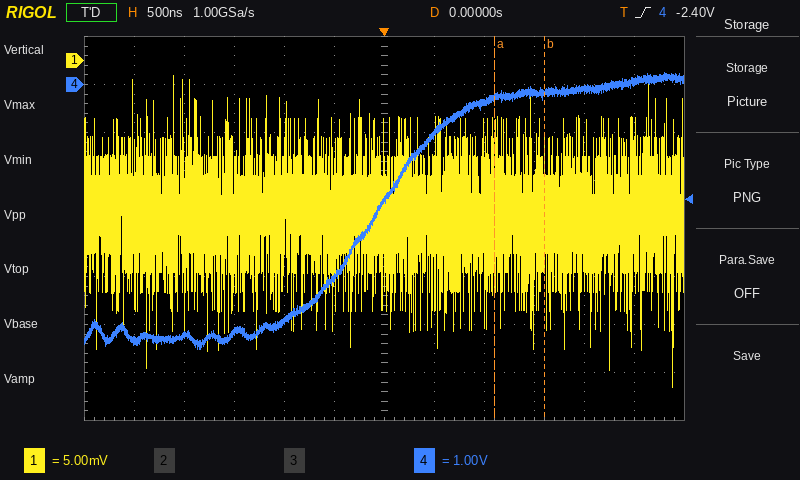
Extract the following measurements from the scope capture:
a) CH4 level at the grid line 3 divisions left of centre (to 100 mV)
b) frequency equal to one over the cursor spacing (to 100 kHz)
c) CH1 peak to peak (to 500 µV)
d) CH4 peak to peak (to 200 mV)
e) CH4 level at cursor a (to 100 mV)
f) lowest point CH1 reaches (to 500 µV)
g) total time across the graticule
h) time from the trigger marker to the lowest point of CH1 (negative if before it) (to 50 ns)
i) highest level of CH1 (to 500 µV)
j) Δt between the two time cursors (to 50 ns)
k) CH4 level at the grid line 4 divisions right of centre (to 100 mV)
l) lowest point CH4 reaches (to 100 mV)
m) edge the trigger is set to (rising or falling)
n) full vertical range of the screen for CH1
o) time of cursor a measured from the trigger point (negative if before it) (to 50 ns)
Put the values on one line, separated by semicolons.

-5.2 V; 2.0 MHz; 32.5 mV; 5.8 V; -300 mV; -34.0 mV; 6 µs; +2.90 µs; -1.5 mV; 500 ns; -100 mV; -5.5 V; rising; 40 mV; +1.10 µs
